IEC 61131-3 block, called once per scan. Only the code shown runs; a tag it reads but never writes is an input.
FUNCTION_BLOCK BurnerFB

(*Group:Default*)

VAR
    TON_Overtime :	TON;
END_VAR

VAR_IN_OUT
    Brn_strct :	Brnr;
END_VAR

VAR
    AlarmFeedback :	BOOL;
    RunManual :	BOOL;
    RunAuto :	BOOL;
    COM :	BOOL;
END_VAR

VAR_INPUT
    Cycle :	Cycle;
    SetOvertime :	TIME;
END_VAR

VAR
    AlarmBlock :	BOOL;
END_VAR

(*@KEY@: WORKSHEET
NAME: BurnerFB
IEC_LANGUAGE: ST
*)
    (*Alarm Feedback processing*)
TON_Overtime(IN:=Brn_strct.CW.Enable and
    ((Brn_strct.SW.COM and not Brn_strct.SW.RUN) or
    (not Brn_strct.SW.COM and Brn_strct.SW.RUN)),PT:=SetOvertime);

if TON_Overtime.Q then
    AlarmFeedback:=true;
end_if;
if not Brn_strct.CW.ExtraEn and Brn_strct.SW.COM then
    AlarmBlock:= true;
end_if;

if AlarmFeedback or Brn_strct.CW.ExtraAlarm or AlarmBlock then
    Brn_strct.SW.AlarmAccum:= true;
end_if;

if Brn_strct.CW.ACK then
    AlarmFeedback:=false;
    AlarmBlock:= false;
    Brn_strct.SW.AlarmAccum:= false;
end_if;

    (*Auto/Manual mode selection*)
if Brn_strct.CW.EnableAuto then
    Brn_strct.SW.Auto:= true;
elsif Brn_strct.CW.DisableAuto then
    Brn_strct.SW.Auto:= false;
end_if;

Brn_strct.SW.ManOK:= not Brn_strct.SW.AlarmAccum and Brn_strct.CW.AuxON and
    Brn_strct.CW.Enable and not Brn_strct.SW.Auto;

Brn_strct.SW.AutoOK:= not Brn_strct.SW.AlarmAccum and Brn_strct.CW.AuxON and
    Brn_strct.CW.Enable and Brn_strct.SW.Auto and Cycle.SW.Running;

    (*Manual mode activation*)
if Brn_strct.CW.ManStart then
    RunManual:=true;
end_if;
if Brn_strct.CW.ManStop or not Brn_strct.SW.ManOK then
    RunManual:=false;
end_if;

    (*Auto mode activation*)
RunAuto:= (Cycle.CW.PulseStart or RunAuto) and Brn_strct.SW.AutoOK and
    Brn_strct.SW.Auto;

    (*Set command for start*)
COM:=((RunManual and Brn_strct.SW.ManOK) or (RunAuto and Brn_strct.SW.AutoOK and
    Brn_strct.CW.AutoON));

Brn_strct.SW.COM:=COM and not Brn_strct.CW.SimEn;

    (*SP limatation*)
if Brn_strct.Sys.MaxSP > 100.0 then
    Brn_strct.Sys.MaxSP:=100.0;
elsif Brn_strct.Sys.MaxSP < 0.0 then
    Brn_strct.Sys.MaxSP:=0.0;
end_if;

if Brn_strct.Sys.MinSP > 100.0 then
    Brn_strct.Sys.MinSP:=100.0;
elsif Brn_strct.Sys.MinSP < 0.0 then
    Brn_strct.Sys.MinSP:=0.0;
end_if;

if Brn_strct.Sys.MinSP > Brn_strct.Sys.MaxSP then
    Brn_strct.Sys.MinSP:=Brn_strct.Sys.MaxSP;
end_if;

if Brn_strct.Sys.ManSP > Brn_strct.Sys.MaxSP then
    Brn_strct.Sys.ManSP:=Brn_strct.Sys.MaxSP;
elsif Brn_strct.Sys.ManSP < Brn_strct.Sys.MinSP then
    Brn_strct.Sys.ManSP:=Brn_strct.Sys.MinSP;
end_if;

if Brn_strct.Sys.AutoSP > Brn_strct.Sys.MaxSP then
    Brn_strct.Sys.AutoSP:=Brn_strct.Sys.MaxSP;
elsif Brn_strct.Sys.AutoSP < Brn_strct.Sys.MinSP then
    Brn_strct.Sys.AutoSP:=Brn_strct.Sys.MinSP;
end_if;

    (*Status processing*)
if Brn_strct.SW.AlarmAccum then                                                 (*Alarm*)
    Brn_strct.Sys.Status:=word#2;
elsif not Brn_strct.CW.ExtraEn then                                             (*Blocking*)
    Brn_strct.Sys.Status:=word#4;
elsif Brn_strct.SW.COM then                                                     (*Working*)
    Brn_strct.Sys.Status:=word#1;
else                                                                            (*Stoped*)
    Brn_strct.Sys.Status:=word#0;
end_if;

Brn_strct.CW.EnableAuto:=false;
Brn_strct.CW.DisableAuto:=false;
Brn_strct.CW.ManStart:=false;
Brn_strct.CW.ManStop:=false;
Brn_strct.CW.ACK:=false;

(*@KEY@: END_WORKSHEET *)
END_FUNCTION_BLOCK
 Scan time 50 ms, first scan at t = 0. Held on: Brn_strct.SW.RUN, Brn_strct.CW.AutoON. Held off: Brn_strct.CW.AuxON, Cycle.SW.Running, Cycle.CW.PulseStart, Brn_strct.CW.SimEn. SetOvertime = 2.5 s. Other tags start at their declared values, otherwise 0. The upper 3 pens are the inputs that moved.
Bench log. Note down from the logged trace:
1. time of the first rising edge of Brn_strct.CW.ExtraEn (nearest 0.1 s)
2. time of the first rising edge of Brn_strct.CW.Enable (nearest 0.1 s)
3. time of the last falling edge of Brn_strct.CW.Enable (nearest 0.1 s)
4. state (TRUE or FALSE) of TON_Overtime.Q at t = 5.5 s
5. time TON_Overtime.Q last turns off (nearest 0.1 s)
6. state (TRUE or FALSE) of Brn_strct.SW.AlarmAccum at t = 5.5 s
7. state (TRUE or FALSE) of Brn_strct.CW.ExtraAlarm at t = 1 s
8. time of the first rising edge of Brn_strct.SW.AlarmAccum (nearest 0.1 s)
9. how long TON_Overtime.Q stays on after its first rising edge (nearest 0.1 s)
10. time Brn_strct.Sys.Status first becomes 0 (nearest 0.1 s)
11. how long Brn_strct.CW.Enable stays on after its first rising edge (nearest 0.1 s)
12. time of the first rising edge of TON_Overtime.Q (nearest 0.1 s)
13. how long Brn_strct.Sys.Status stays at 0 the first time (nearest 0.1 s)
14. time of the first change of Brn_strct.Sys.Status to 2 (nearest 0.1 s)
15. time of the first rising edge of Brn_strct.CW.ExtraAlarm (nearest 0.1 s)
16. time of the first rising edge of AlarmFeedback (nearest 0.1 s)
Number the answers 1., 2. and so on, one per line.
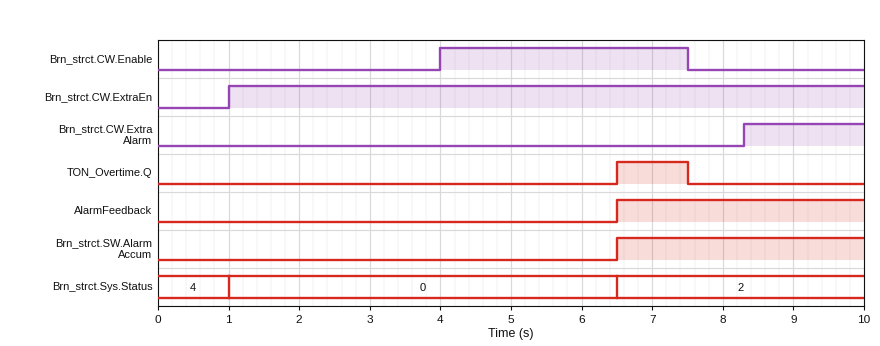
1. 1.0 s
2. 4.0 s
3. 7.5 s
4. FALSE
5. 7.5 s
6. FALSE
7. FALSE
8. 6.5 s
9. 1.0 s
10. 1.0 s
11. 3.5 s
12. 6.5 s
13. 5.5 s
14. 6.5 s
15. 8.3 s
16. 6.5 s
